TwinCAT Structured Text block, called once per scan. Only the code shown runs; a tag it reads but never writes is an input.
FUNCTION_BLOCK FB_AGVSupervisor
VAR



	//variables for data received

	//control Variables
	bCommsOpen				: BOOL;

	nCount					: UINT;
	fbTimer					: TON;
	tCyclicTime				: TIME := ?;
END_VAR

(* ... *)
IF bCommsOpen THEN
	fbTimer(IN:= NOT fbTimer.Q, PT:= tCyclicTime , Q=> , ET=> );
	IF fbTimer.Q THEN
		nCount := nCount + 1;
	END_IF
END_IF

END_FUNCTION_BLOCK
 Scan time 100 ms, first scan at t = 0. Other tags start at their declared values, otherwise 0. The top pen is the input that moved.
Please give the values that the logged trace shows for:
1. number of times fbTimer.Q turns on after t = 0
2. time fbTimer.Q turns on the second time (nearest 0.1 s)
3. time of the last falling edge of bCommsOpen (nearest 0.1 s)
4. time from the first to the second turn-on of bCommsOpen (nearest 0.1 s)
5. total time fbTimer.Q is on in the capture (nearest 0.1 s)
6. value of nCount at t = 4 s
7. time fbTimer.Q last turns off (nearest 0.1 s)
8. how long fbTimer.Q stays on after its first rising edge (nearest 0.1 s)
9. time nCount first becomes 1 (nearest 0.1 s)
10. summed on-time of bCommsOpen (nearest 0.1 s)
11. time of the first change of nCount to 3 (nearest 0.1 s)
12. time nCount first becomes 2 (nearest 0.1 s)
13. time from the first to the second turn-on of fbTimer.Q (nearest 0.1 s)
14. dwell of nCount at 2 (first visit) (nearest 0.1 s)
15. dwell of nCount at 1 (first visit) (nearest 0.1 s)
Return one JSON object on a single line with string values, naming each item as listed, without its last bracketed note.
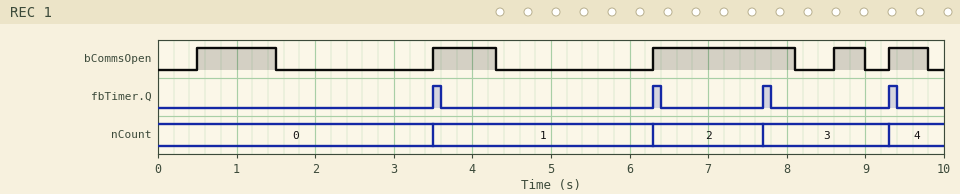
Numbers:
{"number of times fbTimer.Q turns on after t = 0": "4", "time fbTimer.Q turns on the second time": "6.3 s", "time of the last falling edge of bCommsOpen": "9.8 s", "time from the first to the second turn-on of bCommsOpen": "3.0 s", "total time fbTimer.Q is on in the capture": "0.4 s", "value of nCount at t = 4 s": "1", "time fbTimer.Q last turns off": "9.4 s", "how long fbTimer.Q stays on after its first rising edge": "0.1 s", "time nCount first becomes 1": "3.5 s", "summed on-time of bCommsOpen": "4.5 s", "time of the first change of nCount to 3": "7.7 s", "time nCount first becomes 2": "6.3 s", "time from the first to the second turn-on of fbTimer.Q": "2.8 s", "dwell of nCount at 2 (first visit)": "1.4 s", "dwell of nCount at 1 (first visit)": "2.8 s"}
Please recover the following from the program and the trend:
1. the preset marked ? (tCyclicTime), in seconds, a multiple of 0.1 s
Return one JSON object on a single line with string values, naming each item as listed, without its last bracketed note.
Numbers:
{"the preset marked ? (tCyclicTime), in seconds, a multiple of 0.1 s": "1.2 s"}
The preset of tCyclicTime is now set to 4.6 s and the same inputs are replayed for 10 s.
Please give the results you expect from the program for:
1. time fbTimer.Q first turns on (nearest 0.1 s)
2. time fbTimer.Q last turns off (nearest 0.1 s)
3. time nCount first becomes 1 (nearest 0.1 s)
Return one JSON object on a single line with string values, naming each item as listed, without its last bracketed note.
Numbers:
{"time fbTimer.Q first turns on": "6.3 s", "time fbTimer.Q last turns off": "6.4 s", "time nCount first becomes 1": "6.3 s"}
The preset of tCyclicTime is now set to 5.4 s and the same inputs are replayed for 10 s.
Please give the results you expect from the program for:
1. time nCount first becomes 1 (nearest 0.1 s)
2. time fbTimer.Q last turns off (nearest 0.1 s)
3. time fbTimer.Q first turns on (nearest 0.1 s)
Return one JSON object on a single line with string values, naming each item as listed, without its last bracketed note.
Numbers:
{"time nCount first becomes 1": "6.3 s", "time fbTimer.Q last turns off": "6.4 s", "time fbTimer.Q first turns on": "6.3 s"}
